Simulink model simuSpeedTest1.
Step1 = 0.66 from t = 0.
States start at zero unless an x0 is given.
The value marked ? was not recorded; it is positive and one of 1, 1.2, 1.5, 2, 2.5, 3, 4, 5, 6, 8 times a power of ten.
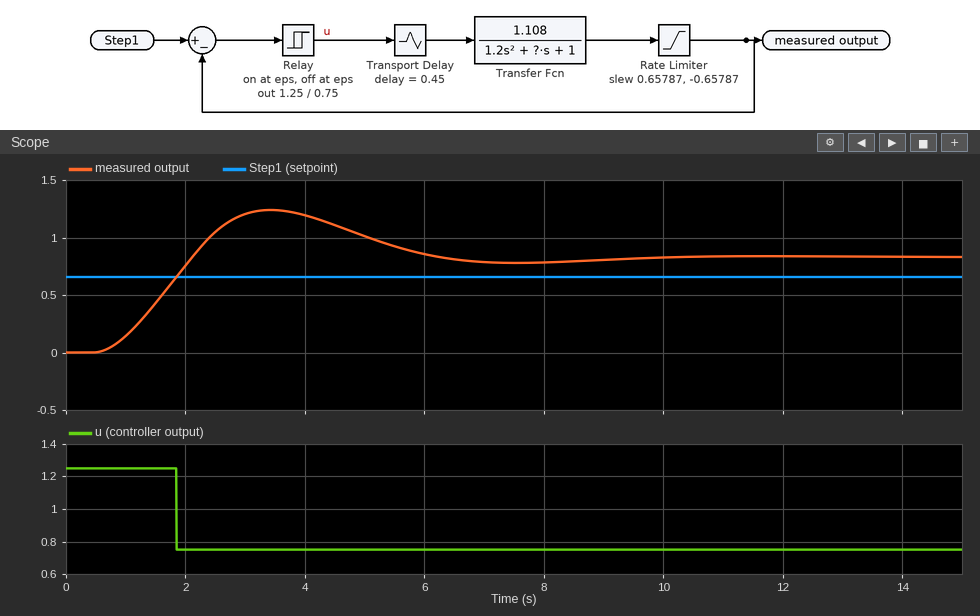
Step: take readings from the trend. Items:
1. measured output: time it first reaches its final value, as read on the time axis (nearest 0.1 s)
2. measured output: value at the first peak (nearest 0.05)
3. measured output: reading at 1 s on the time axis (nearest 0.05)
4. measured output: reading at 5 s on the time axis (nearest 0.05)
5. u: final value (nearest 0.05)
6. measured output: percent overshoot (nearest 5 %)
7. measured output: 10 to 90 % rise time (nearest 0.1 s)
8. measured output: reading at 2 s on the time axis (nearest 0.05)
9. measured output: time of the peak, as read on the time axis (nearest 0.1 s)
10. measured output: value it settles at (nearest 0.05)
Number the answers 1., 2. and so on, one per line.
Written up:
1. 2.1 s
2. 1.25
3. 0.15
4. 1.00
5. 0.75
6. 50 %
7. 1.1 s
8. 0.75
9. 3.4 s
10. 0.85
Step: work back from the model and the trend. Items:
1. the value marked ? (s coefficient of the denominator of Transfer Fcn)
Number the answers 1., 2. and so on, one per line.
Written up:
1. 1.2
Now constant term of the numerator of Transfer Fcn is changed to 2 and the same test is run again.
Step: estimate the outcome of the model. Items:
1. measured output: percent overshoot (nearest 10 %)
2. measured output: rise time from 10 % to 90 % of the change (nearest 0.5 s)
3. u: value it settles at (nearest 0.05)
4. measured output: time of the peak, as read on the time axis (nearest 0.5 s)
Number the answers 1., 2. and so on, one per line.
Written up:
1. 40 %
2. 2.0 s
3. 0.75
4. 4.0 s
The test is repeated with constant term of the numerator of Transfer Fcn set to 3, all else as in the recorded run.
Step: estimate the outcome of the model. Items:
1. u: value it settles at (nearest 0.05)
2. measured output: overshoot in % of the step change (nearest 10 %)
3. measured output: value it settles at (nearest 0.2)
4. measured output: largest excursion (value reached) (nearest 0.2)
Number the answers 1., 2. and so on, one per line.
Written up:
1. 0.75
2. 20 %
3. 2.2
4. 2.8
